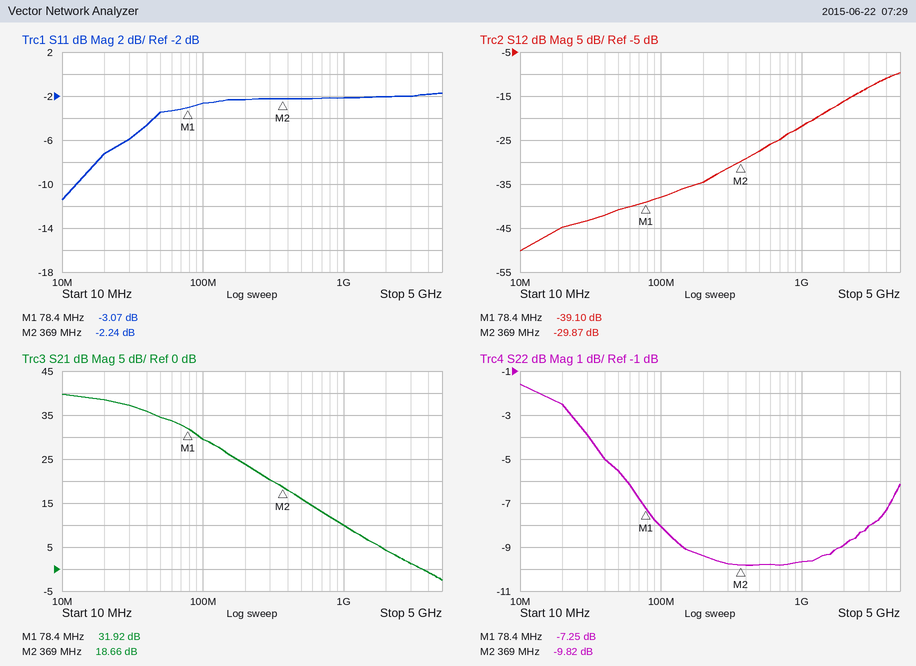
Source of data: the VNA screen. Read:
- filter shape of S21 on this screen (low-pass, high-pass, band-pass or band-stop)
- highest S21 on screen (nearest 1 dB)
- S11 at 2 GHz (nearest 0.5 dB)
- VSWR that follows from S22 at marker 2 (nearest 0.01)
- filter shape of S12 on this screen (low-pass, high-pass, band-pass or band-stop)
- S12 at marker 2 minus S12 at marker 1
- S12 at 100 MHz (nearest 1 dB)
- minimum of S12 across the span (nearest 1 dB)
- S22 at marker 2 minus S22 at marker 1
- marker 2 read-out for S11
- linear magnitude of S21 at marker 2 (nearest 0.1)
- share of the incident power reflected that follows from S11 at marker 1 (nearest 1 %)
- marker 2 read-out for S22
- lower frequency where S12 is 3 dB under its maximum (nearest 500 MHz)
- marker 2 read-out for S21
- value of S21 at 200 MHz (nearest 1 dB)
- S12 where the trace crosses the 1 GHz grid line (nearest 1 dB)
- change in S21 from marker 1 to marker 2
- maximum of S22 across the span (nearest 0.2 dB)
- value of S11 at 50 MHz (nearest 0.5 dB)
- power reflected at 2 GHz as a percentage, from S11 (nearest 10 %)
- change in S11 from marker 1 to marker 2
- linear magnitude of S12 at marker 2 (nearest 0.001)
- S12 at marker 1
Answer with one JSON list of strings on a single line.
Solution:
["low-pass", "40 dB", "-2.0 dB", "1.95", "high-pass", "9.23 dB", "-38 dB", "-50 dB", "-2.57 dB", "-2.24 dB", "8.6", "49 %", "-9.82 dB", "3.0 GHz", "18.66 dB", "24 dB", "-22 dB", "-13.26 dB", "-1.6 dB", "-3.5 dB", "60 %", "0.83 dB", "0.032", "-39.10 dB"]
